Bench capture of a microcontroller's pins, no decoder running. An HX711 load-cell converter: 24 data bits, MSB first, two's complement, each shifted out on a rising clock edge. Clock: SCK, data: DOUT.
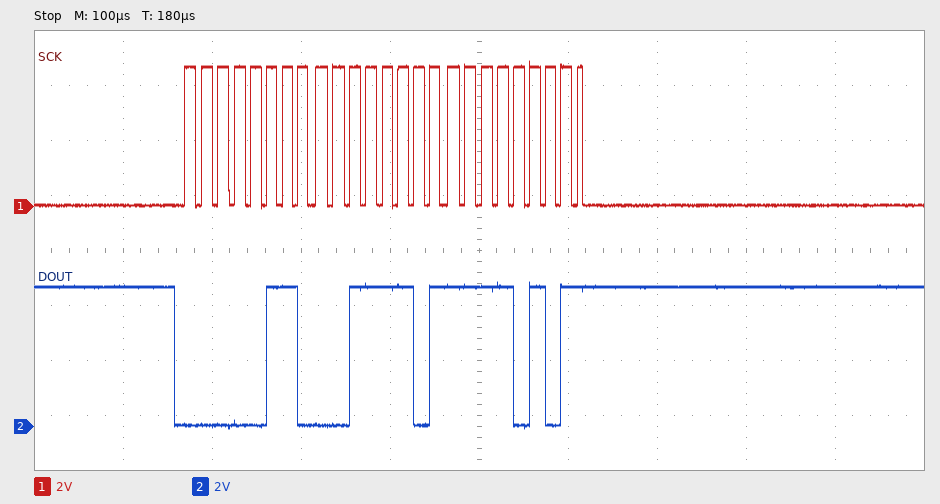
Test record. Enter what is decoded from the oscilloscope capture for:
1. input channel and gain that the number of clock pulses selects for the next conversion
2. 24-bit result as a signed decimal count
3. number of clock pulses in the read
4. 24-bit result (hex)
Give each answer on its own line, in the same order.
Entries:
channel A, gain 128
409077
25
0x063DF5
